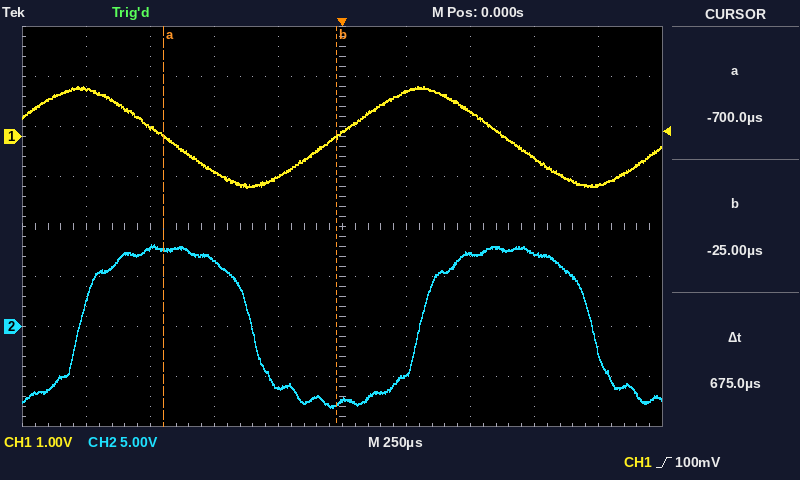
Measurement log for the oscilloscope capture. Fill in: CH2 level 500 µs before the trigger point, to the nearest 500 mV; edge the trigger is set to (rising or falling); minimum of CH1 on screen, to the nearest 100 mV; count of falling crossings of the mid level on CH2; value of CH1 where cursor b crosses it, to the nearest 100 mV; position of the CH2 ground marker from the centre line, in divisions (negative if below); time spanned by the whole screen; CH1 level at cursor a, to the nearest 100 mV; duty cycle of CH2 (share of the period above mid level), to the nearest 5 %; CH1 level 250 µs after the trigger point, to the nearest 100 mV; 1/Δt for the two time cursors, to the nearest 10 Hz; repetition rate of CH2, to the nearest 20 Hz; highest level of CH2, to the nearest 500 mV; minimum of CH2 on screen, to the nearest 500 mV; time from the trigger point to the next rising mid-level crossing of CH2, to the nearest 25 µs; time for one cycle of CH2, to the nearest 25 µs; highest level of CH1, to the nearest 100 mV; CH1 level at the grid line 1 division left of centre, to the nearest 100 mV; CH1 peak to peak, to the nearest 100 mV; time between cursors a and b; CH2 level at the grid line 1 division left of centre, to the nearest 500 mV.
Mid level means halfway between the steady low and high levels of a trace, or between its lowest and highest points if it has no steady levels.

6.5 V
rising
-1.0 V
2
0.0 V
-2.0 div
2.5 ms
0.0 V
50 %
900 mV
1.48 kHz
760 Hz
8.0 V
-8.0 V
300 µs
1.325 ms
1.0 V
-800 mV
2.0 V
675 µs
-6.0 V
